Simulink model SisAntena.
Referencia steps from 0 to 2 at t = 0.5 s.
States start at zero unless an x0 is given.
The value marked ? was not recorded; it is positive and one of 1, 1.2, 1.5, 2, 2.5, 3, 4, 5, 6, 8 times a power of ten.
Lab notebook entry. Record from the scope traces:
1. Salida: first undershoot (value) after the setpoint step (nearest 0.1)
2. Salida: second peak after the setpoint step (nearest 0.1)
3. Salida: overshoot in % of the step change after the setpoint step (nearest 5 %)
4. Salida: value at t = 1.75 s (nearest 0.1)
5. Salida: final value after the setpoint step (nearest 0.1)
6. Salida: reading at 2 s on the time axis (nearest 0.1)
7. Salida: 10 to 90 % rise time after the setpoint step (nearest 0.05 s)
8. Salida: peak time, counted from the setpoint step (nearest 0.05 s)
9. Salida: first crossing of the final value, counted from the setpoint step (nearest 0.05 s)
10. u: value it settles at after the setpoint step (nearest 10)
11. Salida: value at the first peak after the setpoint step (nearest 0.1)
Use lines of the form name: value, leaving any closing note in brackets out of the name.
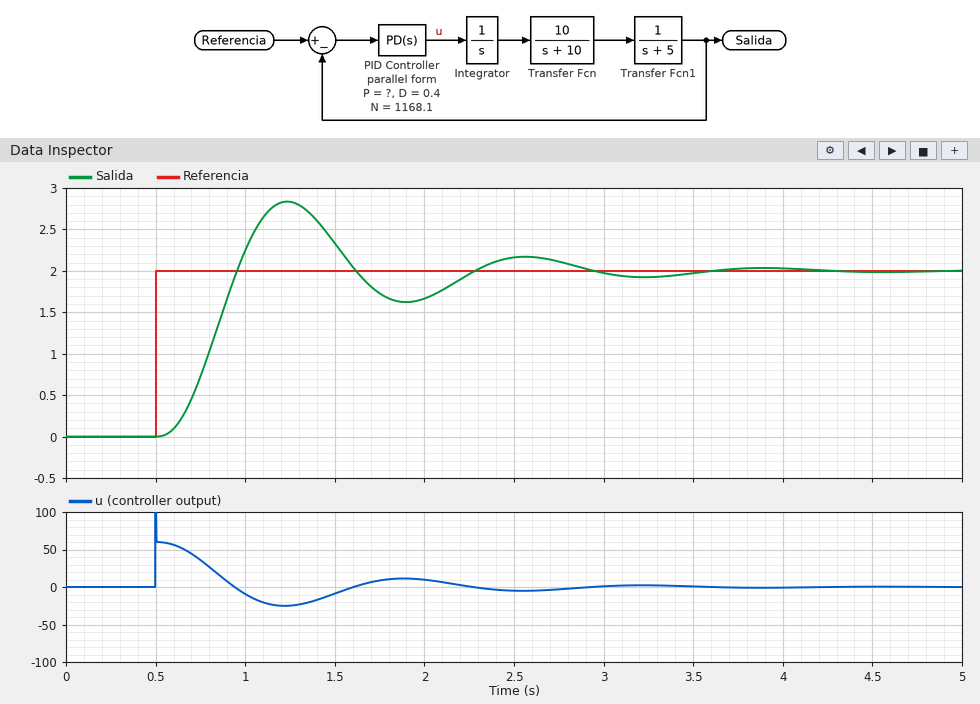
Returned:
Salida: first undershoot (value) after the setpoint step: 1.6
Salida: second peak after the setpoint step: 2.2
Salida: overshoot in % of the step change after the setpoint step: 40 %
Salida: value at t = 1.75 s: 1.7
Salida: final value after the setpoint step: 2.0
Salida: reading at 2 s on the time axis: 1.7
Salida: 10 to 90 % rise time after the setpoint step: 0.30 s
Salida: peak time, counted from the setpoint step: 0.75 s
Salida: first crossing of the final value, counted from the setpoint step: 0.45 s
u: value it settles at after the setpoint step: 0
Salida: value at the first peak after the setpoint step: 2.8
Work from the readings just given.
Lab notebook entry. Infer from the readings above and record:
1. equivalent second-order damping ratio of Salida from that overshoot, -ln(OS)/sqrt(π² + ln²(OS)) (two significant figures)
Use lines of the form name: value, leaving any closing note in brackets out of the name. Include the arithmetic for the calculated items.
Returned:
equivalent second-order damping ratio of Salida from that overshoot, -ln(OS)/sqrt(π² + ln²(OS)): ln(0.4) = -0.916; 0.916 / sqrt(9.870 + 0.840) = 0.28
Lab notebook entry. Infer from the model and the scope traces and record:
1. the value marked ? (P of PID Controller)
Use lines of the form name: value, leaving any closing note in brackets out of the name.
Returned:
the value marked ?: 30
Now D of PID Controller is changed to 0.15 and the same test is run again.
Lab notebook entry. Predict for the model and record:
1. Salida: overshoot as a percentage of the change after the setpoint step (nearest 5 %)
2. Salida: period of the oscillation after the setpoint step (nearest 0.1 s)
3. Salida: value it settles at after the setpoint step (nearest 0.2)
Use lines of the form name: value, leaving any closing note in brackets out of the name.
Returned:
Salida: overshoot as a percentage of the change after the setpoint step: 45 %
Salida: period of the oscillation after the setpoint step: 1.3 s
Salida: value it settles at after the setpoint step: 2.0
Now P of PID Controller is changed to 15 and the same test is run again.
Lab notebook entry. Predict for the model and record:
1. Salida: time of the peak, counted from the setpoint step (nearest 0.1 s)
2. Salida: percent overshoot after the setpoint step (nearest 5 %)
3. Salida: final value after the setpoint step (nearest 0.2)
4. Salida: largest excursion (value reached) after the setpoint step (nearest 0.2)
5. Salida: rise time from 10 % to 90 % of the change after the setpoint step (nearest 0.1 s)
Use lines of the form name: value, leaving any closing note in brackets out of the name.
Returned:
Salida: time of the peak, counted from the setpoint step: 1.1 s
Salida: percent overshoot after the setpoint step: 15 %
Salida: final value after the setpoint step: 2.0
Salida: largest excursion (value reached) after the setpoint step: 2.4
Salida: rise time from 10 % to 90 % of the change after the setpoint step: 0.5 s
